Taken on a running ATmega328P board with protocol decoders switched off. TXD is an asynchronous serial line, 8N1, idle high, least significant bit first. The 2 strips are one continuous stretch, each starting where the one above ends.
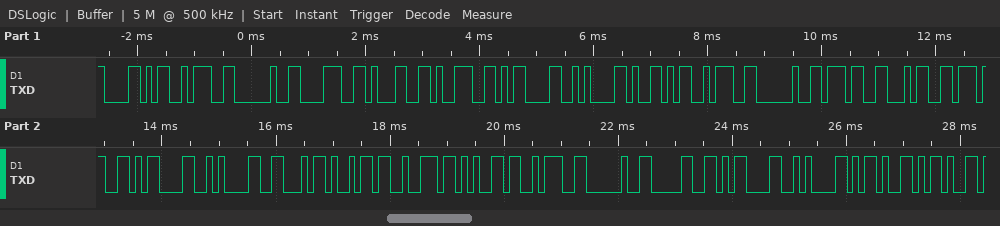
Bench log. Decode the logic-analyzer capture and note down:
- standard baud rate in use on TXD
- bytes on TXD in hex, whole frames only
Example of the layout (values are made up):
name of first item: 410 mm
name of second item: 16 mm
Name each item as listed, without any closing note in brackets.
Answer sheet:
standard baud rate in use on TXD: 9600 baud
bytes on TXD in hex, whole frames only: 0x58 0x3A 0x20 0x38 0x31 0x39 0x0D 0x0A 0x59 0x3A 0x20 0x37 0x34 0x37 0x0D 0x0A 0x46 0x69 0x72 0x65 0x3A 0x20 0x30 0x0D 0x0A 0x2D 0x2D
